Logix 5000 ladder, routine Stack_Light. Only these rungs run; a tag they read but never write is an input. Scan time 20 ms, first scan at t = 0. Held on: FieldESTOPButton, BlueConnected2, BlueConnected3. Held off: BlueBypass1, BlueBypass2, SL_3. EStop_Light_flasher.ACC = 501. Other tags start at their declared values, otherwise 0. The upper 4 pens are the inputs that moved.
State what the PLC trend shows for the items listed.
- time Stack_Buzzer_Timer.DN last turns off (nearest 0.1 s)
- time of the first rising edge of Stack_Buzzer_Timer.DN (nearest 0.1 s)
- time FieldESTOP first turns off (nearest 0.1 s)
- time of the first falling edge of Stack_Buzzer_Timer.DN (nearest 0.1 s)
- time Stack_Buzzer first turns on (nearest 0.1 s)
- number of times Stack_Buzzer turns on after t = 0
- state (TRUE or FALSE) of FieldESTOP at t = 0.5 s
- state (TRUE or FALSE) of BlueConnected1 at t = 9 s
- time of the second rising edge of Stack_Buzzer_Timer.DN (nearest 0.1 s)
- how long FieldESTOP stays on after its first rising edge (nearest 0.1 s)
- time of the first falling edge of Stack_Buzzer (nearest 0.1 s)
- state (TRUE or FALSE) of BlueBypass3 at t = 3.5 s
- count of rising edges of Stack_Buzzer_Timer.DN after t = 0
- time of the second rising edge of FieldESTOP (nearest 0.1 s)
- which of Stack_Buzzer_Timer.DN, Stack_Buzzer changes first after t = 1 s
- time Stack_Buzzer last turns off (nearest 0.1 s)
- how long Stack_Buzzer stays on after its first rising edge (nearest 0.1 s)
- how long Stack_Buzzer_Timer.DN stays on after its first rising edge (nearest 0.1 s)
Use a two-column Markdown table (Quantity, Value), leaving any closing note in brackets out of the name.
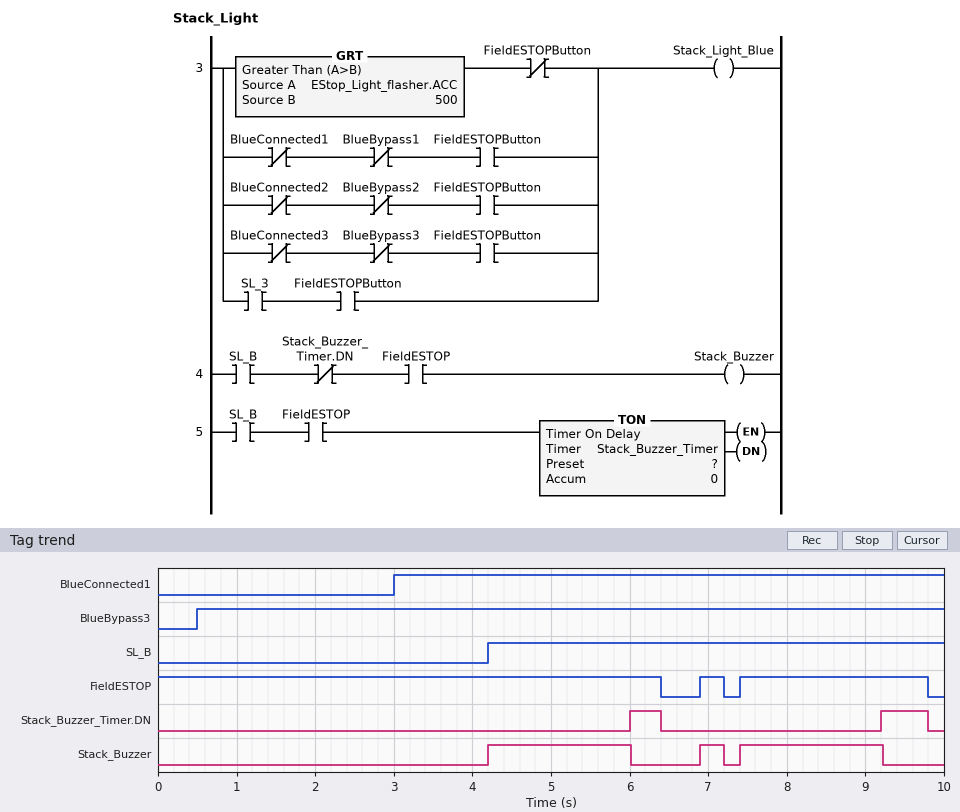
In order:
| Quantity | Value |
|---|---|
| time Stack_Buzzer_Timer.DN last turns off | 9.8 s |
| time of the first rising edge of Stack_Buzzer_Timer.DN | 6.0 s |
| time FieldESTOP first turns off | 6.4 s |
| time of the first falling edge of Stack_Buzzer_Timer.DN | 6.4 s |
| time Stack_Buzzer first turns on | 4.2 s |
| number of times Stack_Buzzer turns on after t = 0 | 3 |
| state (TRUE or FALSE) of FieldESTOP at t = 0.5 s | TRUE |
| state (TRUE or FALSE) of BlueConnected1 at t = 9 s | TRUE |
| time of the second rising edge of Stack_Buzzer_Timer.DN | 9.2 s |
| how long FieldESTOP stays on after its first rising edge | 0.3 s |
| time of the first falling edge of Stack_Buzzer | 6.0 s |
| state (TRUE or FALSE) of BlueBypass3 at t = 3.5 s | TRUE |
| count of rising edges of Stack_Buzzer_Timer.DN after t = 0 | 2 |
| time of the second rising edge of FieldESTOP | 7.4 s |
| which of Stack_Buzzer_Timer.DN, Stack_Buzzer changes first after t = 1 s | Stack_Buzzer |
| time Stack_Buzzer last turns off | 9.2 s |
| how long Stack_Buzzer stays on after its first rising edge | 1.8 s |
| how long Stack_Buzzer_Timer.DN stays on after its first rising edge | 0.4 s |
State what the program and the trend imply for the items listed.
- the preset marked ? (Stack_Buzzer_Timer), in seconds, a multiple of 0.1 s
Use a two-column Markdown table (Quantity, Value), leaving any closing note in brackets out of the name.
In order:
| Quantity | Value |
|---|---|
| the preset marked ? (Stack_Buzzer_Timer), in seconds, a multiple of 0.1 s | 1.8 s |
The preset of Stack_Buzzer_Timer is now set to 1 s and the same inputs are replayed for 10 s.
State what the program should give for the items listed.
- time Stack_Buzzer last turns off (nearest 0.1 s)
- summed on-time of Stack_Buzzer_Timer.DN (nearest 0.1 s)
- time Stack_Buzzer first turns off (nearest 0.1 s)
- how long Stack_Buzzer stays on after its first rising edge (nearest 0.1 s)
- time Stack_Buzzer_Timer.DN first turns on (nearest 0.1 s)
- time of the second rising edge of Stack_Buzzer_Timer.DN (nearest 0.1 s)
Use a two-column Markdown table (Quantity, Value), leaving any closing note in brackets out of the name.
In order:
| Quantity | Value |
|---|---|
| time Stack_Buzzer last turns off | 8.4 s |
| summed on-time of Stack_Buzzer_Timer.DN | 2.6 s |
| time Stack_Buzzer first turns off | 5.2 s |
| how long Stack_Buzzer stays on after its first rising edge | 1.0 s |
| time Stack_Buzzer_Timer.DN first turns on | 5.2 s |
| time of the second rising edge of Stack_Buzzer_Timer.DN | 8.4 s |
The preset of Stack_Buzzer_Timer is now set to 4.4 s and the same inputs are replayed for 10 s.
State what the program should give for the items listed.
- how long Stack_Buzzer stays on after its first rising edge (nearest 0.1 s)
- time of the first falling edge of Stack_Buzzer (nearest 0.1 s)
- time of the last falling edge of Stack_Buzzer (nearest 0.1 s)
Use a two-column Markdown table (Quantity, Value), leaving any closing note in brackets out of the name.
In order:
| Quantity | Value |
|---|---|
| how long Stack_Buzzer stays on after its first rising edge | 2.2 s |
| time of the first falling edge of Stack_Buzzer | 6.4 s |
| time of the last falling edge of Stack_Buzzer | 9.8 s |
